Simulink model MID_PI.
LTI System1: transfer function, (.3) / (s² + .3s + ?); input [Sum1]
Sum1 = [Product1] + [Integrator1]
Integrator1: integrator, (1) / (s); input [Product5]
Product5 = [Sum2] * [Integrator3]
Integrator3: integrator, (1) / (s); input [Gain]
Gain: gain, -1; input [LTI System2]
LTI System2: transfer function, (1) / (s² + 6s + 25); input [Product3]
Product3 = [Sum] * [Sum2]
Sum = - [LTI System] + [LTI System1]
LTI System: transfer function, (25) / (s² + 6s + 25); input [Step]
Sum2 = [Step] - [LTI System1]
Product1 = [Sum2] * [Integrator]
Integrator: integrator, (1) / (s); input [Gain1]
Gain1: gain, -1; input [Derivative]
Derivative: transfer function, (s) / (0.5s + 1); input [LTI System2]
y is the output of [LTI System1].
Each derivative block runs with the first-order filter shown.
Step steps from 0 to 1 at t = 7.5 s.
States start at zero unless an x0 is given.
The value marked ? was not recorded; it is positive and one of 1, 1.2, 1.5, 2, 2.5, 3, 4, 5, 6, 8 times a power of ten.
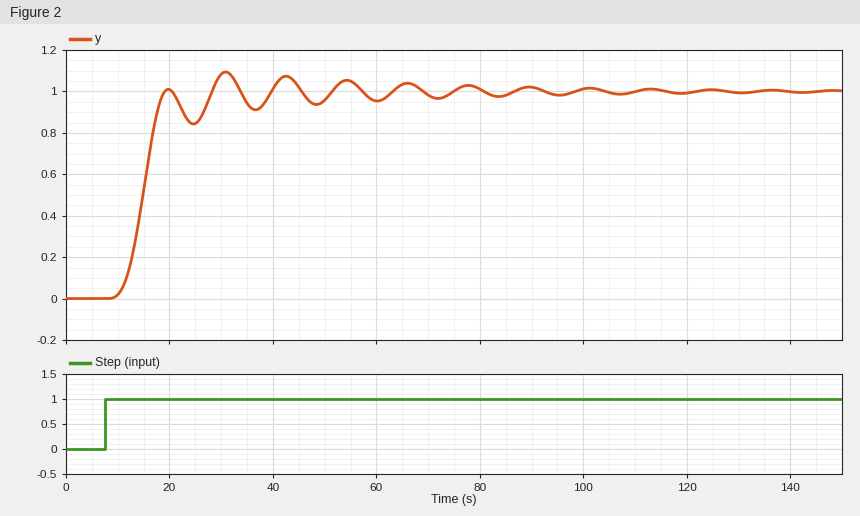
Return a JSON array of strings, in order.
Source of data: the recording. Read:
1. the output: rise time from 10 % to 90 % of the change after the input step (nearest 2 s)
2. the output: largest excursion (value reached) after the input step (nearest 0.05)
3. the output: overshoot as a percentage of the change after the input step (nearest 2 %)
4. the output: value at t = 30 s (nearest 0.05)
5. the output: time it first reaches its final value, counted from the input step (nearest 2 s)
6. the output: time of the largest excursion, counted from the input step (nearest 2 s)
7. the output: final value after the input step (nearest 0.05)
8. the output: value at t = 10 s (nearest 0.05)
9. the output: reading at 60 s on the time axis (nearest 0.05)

["6 s", "1.10", "10 %", "1.10", "12 s", "24 s", "1.00", "0.00", "0.95"]
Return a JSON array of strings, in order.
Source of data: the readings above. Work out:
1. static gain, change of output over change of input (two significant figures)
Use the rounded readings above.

["1.0"]
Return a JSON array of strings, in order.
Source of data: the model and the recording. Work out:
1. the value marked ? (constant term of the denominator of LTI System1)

["0.3"]
